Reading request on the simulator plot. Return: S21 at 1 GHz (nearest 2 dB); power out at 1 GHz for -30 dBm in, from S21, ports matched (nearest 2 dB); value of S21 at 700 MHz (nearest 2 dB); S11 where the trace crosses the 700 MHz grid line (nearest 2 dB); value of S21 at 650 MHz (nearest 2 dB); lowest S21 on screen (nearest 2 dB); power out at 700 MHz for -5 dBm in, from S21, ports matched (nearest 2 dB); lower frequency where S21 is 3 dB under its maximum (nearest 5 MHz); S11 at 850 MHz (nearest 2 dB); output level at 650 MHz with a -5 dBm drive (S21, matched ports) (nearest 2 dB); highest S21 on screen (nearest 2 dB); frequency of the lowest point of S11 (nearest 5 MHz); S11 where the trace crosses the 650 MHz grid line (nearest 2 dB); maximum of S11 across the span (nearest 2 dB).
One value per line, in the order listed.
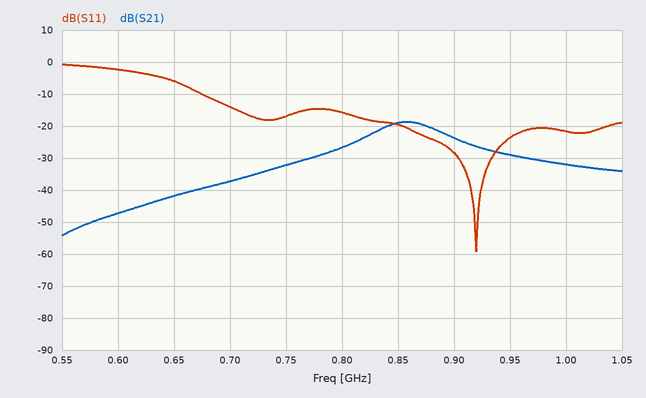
-32 dB
-62 dBm
-38 dB
-14 dB
-42 dB
-54 dB
-42 dBm
830 MHz
-20 dB
-46 dBm
-18 dB
920 MHz
-6 dB
0 dB
